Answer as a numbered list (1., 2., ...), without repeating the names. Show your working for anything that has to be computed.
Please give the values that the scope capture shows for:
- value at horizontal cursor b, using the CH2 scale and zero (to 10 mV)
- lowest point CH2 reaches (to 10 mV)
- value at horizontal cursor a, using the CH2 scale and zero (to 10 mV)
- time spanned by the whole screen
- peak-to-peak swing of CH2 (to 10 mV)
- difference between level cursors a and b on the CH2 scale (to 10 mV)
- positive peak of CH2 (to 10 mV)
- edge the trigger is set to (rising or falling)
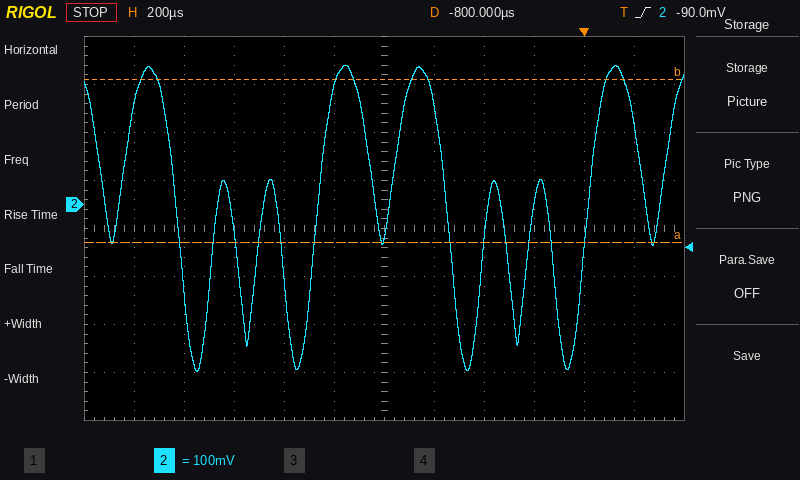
1. 260 mV
2. -350 mV
3. -80 mV
4. 2.4 ms
5. 290 mV − (-350 mV) = 640 mV
6. 340 mV
7. 290 mV
8. rising
